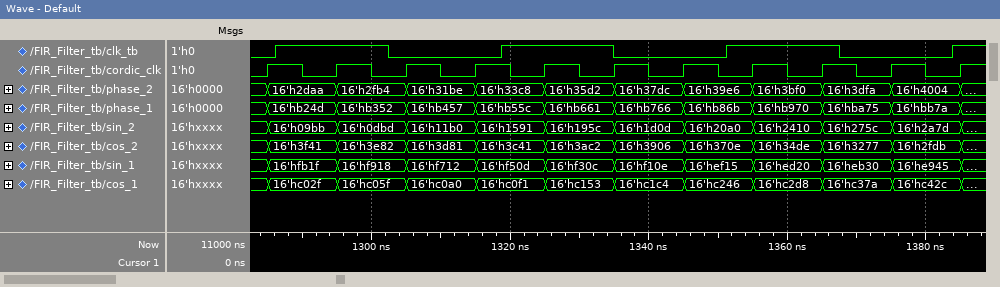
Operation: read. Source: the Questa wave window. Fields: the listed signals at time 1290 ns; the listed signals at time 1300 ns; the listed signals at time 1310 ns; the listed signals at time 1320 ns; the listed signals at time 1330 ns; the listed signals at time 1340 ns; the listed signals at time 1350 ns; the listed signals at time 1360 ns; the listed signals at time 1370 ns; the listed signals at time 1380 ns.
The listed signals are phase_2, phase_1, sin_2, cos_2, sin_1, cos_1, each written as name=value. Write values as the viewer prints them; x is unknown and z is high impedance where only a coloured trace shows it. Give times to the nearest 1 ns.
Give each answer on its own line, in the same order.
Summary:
phase_2=16'h2daa, phase_1=16'hb24d, sin_2=16'h09bb, cos_2=16'h3f41, sin_1=16'hfb1f, cos_1=16'hc02f
phase_2=16'h2fb4, phase_1=16'hb352, sin_2=16'h0dbd, cos_2=16'h3e82, sin_1=16'hf918, cos_1=16'hc05f
phase_2=16'h31be, phase_1=16'hb457, sin_2=16'h11b0, cos_2=16'h3d81, sin_1=16'hf712, cos_1=16'hc0a0
phase_2=16'h33c8, phase_1=16'hb55c, sin_2=16'h1591, cos_2=16'h3c41, sin_1=16'hf50d, cos_1=16'hc0f1
phase_2=16'h35d2, phase_1=16'hb661, sin_2=16'h195c, cos_2=16'h3ac2, sin_1=16'hf30c, cos_1=16'hc153
phase_2=16'h37dc, phase_1=16'hb766, sin_2=16'h1d0d, cos_2=16'h3906, sin_1=16'hf10e, cos_1=16'hc1c4
phase_2=16'h39e6, phase_1=16'hb86b, sin_2=16'h20a0, cos_2=16'h370e, sin_1=16'hef15, cos_1=16'hc246
phase_2=16'h3bf0, phase_1=16'hb970, sin_2=16'h2410, cos_2=16'h34de, sin_1=16'hed20, cos_1=16'hc2d8
phase_2=16'h3dfa, phase_1=16'hba75, sin_2=16'h275c, cos_2=16'h3277, sin_1=16'heb30, cos_1=16'hc37a
phase_2=16'h4004, phase_1=16'hbb7a, sin_2=16'h2a7d, cos_2=16'h2fdb, sin_1=16'he945, cos_1=16'hc42c
